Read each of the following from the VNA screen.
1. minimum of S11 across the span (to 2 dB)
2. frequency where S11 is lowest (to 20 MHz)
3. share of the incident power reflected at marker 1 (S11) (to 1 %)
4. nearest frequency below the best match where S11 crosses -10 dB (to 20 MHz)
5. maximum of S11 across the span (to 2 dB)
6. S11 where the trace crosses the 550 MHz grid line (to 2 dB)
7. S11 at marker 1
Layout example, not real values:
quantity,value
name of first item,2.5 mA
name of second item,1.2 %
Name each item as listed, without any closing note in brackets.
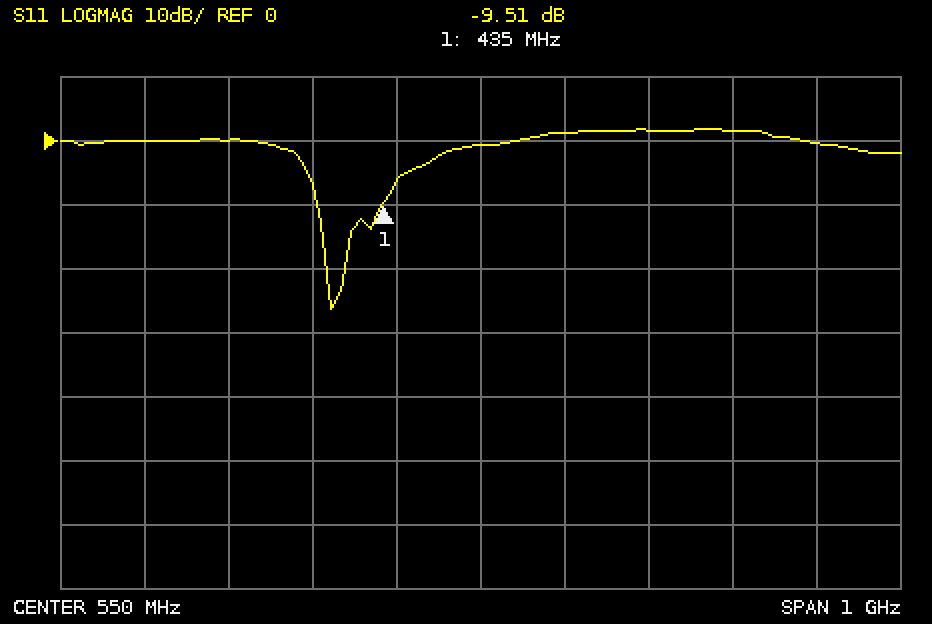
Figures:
quantity,value
minimum of S11 across the span,-26 dB
frequency where S11 is lowest,380 MHz
share of the incident power reflected at marker 1 (S11),11 %
nearest frequency below the best match where S11 crosses -10 dB,360 MHz
maximum of S11 across the span,2 dB
S11 where the trace crosses the 550 MHz grid line,0 dB
S11 at marker 1,-9.51 dB
